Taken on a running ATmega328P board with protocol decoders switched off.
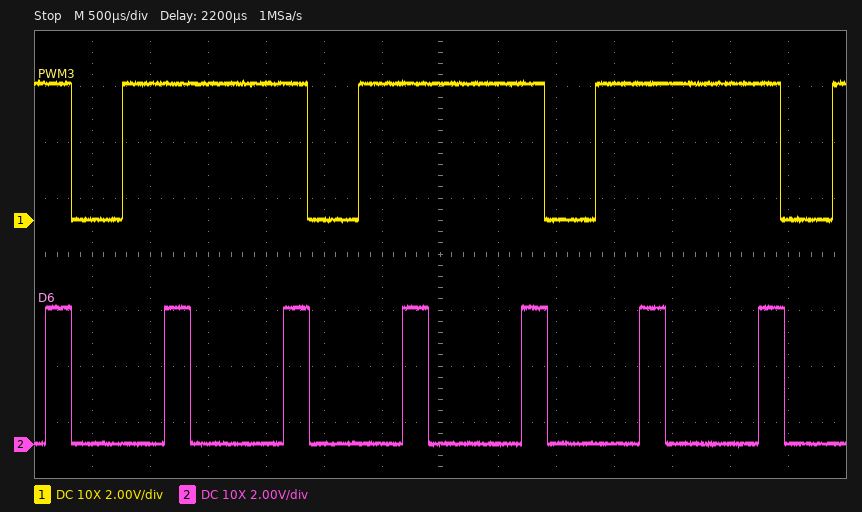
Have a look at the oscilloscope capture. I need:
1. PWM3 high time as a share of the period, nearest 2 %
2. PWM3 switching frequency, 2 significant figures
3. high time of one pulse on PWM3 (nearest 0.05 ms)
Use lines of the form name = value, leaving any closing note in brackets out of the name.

PWM3 high time as a share of the period, nearest 2 % = 78 %
PWM3 switching frequency, 2 significant figures = 490 Hz
high time of one pulse on PWM3 = 1.60 ms
